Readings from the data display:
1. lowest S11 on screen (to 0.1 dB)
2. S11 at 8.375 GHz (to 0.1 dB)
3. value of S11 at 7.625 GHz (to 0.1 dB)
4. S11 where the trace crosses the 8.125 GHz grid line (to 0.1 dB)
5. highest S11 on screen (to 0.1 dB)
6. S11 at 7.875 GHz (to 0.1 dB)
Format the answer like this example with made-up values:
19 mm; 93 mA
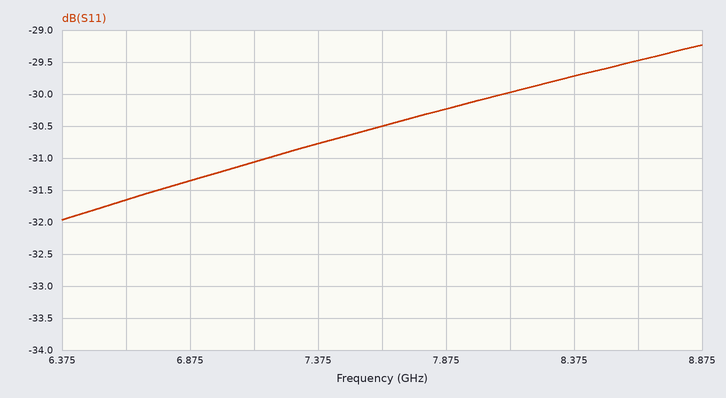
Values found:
-32.0 dB; -29.7 dB; -30.5 dB; -30.0 dB; -29.2 dB; -30.2 dB
